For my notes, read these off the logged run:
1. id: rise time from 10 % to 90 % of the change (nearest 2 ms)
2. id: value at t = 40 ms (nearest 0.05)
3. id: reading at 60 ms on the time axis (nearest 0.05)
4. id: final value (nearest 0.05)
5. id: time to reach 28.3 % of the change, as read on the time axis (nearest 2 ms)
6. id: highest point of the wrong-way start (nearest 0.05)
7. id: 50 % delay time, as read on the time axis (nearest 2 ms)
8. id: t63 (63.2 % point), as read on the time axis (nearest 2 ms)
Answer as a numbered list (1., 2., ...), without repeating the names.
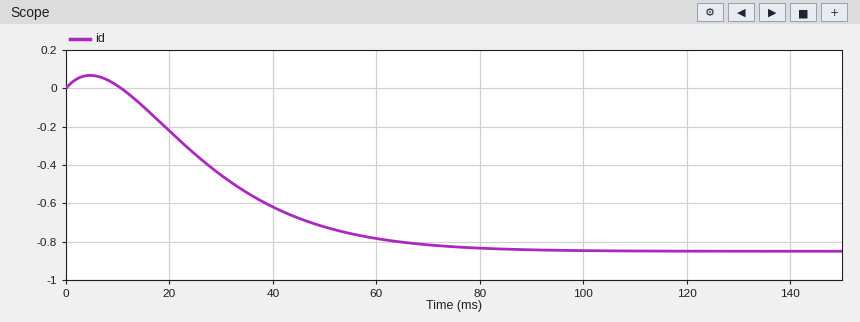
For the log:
1. 42 ms
2. -0.60
3. -0.80
4. -0.85
5. 20 ms
6. 0.05
7. 28 ms
8. 34 ms
